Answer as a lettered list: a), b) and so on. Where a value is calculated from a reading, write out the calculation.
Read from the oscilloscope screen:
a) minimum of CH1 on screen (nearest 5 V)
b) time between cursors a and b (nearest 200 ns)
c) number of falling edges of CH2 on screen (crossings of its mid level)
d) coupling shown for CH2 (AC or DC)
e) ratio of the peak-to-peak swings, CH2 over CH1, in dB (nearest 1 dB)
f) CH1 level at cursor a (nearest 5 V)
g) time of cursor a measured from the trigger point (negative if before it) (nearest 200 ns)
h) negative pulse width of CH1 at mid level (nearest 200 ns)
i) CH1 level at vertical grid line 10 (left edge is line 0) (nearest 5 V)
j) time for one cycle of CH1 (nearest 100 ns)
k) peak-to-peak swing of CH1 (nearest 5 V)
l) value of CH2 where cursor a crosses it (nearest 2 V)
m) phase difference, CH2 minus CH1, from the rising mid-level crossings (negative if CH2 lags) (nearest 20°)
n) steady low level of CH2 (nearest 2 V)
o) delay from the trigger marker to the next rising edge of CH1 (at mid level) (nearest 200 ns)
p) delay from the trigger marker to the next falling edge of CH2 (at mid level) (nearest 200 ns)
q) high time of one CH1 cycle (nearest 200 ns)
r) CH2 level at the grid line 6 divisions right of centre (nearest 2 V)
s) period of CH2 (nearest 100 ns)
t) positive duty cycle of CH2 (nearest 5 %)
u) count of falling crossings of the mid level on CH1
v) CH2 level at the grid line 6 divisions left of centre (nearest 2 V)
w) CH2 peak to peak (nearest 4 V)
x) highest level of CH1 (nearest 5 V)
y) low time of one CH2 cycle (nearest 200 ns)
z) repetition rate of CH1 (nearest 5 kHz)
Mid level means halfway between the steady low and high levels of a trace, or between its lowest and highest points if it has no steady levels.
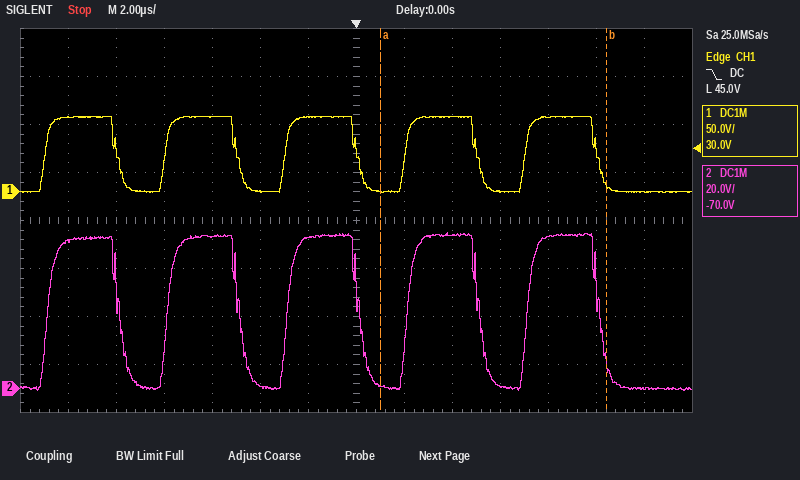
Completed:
a) 0 V
b) 9.4 µs
c) 5
d) DC
e) 20 log10(64 V / 80 V) ≈ -2 dB
f) 0 V
g) +1.0 µs
h) 2.0 µs
i) 0 V
j) 5.0 µs
k) 80 V − (0 V) = 80 V
l) 2 V
m) 0°
n) 0 V
o) 2.0 µs
p) 200 ns
q) 3.0 µs
r) 0 V
s) 5.0 µs
t) 3.0 µs / 5.0 µs ≈ 60 %
u) 5
v) 62 V
w) 64 V
x) 80 V
y) 2.0 µs
z) 1 / 5.0 µs ≈ 200 kHz
